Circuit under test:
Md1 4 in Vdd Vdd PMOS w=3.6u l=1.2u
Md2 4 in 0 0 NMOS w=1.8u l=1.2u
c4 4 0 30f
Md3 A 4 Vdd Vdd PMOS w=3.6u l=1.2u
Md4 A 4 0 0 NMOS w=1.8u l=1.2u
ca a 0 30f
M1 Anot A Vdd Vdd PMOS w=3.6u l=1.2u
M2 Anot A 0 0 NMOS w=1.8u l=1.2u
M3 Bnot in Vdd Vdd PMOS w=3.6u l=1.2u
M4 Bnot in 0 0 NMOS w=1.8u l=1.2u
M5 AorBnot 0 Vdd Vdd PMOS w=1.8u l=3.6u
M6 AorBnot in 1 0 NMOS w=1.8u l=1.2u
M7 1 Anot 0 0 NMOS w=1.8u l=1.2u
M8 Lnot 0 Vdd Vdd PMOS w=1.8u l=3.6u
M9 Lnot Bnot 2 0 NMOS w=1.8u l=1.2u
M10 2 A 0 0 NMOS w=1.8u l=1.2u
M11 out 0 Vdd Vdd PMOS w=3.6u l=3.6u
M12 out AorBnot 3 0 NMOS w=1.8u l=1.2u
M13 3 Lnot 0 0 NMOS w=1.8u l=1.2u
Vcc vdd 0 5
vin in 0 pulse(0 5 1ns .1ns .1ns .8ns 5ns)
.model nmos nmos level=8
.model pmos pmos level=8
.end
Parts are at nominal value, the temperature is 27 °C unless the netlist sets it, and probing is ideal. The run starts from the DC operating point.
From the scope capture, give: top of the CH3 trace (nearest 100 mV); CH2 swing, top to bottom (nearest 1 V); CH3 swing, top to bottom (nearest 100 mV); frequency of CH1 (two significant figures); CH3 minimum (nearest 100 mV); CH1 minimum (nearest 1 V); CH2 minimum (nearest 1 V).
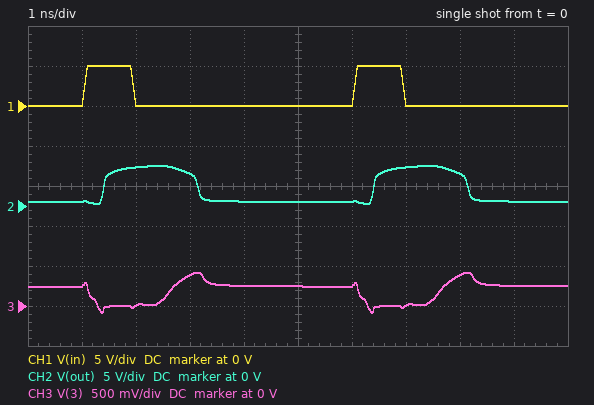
400 mV
5 V
500 mV
200 MHz
-100 mV
0 V
0 V
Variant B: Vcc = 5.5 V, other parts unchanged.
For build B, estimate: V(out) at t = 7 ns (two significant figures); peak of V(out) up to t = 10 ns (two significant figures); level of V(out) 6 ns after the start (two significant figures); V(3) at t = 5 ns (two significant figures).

5.3 V
5.5 V
600 mV
280 mV
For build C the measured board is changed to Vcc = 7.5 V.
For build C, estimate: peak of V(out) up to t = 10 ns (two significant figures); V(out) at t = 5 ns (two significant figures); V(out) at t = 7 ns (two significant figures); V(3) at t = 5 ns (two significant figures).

7.4 V
900 mV
7.2 V
420 mV
